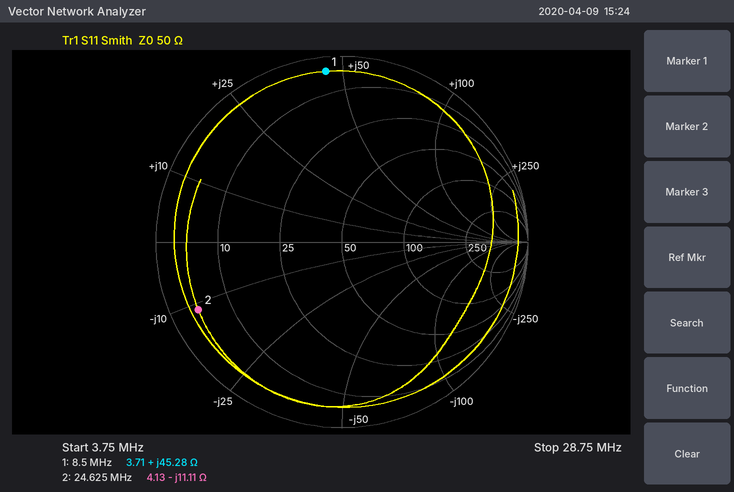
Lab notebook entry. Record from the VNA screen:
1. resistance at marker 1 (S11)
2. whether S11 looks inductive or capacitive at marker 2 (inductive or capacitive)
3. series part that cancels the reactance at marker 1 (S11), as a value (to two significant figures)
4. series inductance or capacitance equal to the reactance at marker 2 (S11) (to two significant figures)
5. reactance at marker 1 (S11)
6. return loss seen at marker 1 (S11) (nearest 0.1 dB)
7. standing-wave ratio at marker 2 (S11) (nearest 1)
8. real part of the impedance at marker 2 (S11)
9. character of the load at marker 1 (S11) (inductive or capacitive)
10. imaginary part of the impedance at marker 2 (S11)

3.71 Ω
capacitive
410 pF
580 pF
+45.28 Ω
0.7 dB
13
4.13 Ω
inductive
-11.11 Ω
